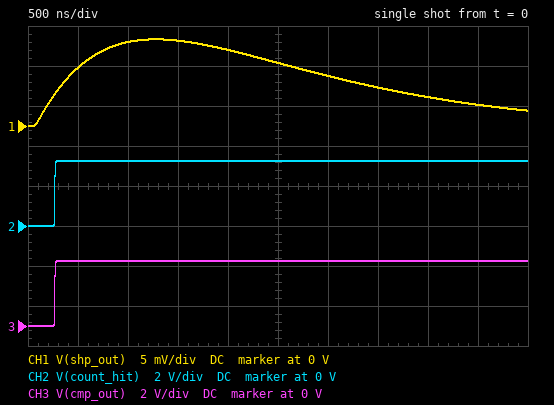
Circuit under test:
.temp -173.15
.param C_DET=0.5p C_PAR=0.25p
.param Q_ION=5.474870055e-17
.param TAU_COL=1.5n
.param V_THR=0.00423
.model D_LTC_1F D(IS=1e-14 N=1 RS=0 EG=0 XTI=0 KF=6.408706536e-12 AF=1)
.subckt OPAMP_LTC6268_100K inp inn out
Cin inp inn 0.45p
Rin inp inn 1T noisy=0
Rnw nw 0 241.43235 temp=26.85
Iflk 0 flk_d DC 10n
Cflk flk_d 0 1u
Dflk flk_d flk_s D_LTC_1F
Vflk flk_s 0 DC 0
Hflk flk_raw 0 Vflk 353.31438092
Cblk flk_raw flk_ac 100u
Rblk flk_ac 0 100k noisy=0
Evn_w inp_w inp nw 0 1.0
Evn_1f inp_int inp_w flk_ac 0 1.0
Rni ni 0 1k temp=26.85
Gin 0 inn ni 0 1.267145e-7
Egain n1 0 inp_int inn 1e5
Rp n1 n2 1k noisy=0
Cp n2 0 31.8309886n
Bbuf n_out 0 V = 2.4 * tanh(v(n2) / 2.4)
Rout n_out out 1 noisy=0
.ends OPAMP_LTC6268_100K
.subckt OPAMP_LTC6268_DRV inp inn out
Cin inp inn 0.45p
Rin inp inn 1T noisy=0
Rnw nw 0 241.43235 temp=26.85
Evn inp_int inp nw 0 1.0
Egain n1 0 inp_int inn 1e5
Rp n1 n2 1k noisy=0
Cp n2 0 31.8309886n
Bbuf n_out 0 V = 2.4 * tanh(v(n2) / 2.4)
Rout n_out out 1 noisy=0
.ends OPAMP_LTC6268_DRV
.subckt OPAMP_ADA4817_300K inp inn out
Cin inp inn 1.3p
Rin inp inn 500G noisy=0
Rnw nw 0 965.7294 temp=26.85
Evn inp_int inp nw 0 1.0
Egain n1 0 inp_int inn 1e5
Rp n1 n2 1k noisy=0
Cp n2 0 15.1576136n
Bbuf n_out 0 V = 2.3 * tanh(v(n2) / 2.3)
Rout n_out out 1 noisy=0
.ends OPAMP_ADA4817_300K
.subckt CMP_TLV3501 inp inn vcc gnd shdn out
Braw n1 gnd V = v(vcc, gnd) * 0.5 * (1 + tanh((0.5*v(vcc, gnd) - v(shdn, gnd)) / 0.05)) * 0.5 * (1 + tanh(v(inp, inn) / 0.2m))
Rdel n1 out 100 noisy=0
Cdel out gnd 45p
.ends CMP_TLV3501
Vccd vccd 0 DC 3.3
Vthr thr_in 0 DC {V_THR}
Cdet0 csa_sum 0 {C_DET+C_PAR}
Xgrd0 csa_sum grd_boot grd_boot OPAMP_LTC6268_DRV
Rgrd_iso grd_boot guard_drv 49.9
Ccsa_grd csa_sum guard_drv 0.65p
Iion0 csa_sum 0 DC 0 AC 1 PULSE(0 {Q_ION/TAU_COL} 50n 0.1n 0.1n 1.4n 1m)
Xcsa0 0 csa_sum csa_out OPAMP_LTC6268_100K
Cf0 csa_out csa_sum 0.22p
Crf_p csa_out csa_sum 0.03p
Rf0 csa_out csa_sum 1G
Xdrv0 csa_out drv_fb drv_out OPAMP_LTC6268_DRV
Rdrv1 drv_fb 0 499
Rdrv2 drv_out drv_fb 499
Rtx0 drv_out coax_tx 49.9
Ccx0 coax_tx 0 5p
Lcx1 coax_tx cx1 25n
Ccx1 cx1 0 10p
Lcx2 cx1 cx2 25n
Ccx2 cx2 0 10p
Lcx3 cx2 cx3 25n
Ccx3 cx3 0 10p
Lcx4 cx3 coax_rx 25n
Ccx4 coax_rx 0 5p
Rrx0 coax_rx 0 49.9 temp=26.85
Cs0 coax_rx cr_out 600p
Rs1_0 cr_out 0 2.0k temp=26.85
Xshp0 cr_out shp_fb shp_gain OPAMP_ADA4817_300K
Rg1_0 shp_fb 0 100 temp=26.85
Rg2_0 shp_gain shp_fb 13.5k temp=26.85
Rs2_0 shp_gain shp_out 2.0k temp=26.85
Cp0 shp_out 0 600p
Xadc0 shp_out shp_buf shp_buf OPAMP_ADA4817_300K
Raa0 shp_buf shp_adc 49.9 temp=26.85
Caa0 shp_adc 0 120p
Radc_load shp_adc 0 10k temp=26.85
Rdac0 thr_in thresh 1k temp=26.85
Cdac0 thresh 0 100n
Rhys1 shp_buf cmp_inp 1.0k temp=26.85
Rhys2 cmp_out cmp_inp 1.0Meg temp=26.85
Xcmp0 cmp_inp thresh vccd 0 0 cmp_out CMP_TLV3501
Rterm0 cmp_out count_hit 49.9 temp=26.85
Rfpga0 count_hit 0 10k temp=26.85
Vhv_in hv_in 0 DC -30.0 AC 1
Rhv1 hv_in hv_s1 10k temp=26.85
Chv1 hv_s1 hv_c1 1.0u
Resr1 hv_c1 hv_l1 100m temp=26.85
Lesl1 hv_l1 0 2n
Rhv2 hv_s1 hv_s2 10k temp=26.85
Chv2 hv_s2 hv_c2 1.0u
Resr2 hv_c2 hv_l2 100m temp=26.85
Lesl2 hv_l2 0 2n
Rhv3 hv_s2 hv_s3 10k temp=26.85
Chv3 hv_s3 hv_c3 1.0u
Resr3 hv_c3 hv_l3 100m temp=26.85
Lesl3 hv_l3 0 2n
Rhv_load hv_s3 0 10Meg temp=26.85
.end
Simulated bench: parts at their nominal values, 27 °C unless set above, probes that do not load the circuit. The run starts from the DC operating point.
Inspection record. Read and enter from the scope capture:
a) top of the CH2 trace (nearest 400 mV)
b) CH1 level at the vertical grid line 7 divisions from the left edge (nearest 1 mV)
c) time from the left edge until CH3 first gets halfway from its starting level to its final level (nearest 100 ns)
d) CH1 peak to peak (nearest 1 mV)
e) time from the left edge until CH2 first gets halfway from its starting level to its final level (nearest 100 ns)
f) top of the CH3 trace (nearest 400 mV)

3.2 V
5 mV
300 ns
11 mV
300 ns
3.2 V
